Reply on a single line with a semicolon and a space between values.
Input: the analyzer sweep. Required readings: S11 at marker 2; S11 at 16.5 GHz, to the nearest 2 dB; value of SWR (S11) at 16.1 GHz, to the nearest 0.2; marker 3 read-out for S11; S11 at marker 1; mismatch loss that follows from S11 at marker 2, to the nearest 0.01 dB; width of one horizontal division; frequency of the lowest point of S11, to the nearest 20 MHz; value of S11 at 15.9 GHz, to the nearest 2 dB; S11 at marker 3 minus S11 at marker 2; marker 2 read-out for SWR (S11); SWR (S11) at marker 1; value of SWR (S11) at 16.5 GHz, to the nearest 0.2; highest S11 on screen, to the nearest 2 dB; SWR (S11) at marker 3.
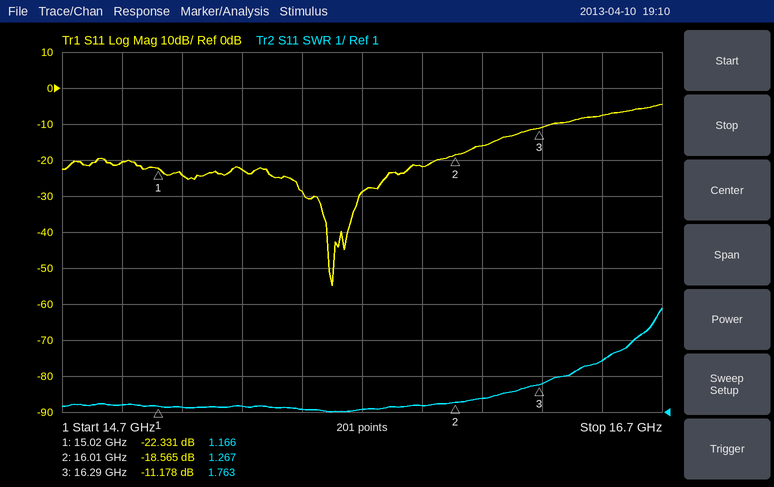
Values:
-18.565 dB; -8 dB; 1.4; -11.178 dB; -22.331 dB; 0.06 dB; 200 MHz; 15.60 GHz; -22 dB; 7.387 dB; 1.267; 1.166; 2.4; -4 dB; 1.763
